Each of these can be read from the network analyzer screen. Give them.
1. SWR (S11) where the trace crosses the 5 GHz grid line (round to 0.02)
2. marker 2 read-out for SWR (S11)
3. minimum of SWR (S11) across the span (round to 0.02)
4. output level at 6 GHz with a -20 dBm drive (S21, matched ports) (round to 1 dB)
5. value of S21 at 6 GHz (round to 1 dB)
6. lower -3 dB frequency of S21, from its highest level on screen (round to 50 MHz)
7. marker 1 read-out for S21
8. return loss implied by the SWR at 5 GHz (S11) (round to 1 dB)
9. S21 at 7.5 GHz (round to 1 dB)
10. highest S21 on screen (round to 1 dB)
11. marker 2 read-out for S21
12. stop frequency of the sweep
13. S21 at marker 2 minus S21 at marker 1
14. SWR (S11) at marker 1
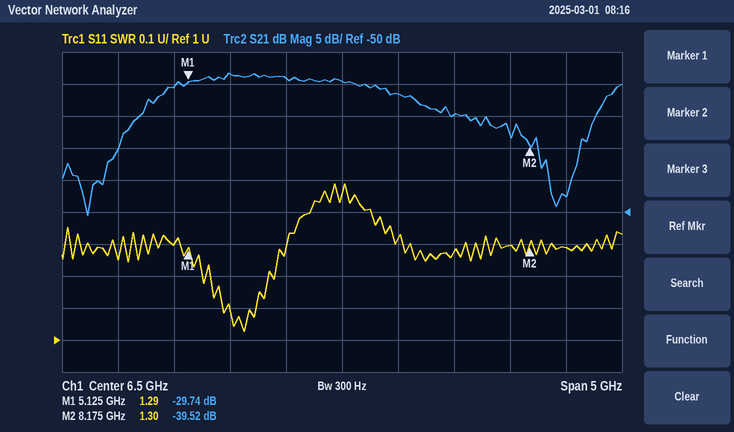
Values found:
1.30
1.30
1.02
-49 dBm
-29 dB
4.90 GHz
-29.74 dB
18 dB
-35 dB
-28 dB
-39.52 dB
9 GHz
-9.78 dB
1.29
